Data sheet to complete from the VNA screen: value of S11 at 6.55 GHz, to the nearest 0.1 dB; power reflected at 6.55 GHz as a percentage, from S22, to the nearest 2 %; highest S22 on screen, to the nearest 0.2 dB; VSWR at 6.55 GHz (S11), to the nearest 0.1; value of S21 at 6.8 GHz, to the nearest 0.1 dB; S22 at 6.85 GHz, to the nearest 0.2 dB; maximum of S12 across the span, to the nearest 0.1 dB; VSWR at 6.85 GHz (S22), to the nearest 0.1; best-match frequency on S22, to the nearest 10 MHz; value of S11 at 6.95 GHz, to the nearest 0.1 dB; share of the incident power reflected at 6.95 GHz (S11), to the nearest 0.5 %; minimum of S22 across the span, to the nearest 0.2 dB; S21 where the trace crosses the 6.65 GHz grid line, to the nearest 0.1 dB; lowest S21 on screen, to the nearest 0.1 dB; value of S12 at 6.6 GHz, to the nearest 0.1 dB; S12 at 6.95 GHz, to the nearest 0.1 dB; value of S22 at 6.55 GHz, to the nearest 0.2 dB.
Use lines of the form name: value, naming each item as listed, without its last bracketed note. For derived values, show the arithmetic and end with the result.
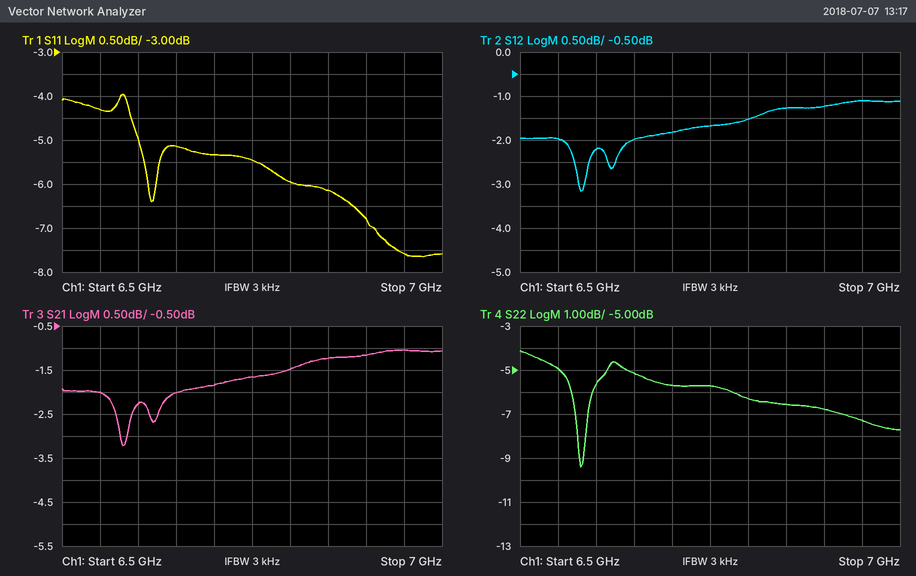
value of S11 at 6.55 GHz, to the nearest 0.1 dB: -4.3 dB
power reflected at 6.55 GHz as a percentage, from S22, to the nearest 2 %: 10^(-5/10) ≈ 32 %
highest S22 on screen, to the nearest 0.2 dB: -4.2 dB
VSWR at 6.55 GHz (S11), to the nearest 0.1: |Γ| = 10^(-4.3/20) = 0.6095; VSWR = (1 + 0.6095)/(1 − 0.6095) ≈ 4.1
value of S21 at 6.8 GHz, to the nearest 0.1 dB: -1.5 dB
S22 at 6.85 GHz, to the nearest 0.2 dB: -6.6 dB
maximum of S12 across the span, to the nearest 0.1 dB: -1.1 dB
VSWR at 6.85 GHz (S22), to the nearest 0.1: |Γ| = 10^(-6.6/20) = 0.4677; VSWR = (1 + 0.4677)/(1 − 0.4677) ≈ 2.8
best-match frequency on S22, to the nearest 10 MHz: 6.58 GHz
value of S11 at 6.95 GHz, to the nearest 0.1 dB: -7.6 dB
share of the incident power reflected at 6.95 GHz (S11), to the nearest 0.5 %: 10^(-7.6/10) ≈ 17.4 %, so 17.5 % to the nearest 0.5 %
minimum of S22 across the span, to the nearest 0.2 dB: -9.4 dB
S21 where the trace crosses the 6.65 GHz grid line, to the nearest 0.1 dB: -2.0 dB
lowest S21 on screen, to the nearest 0.1 dB: -3.2 dB
value of S12 at 6.6 GHz, to the nearest 0.1 dB: -2.2 dB
S12 at 6.95 GHz, to the nearest 0.1 dB: -1.1 dB
value of S22 at 6.55 GHz, to the nearest 0.2 dB: -5.0 dB
